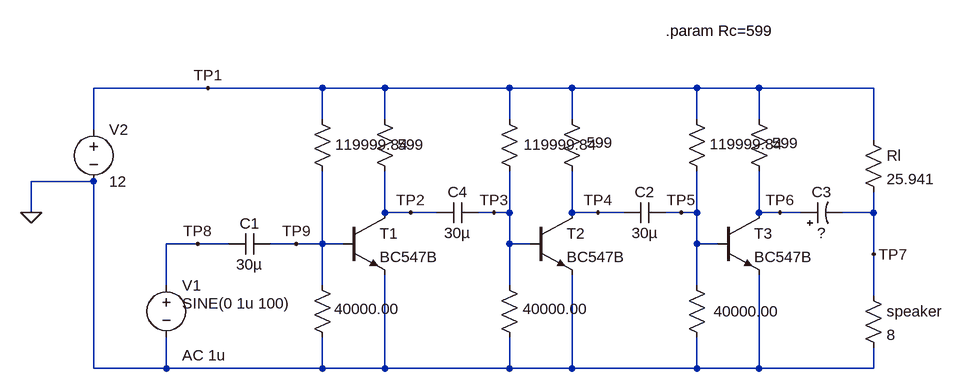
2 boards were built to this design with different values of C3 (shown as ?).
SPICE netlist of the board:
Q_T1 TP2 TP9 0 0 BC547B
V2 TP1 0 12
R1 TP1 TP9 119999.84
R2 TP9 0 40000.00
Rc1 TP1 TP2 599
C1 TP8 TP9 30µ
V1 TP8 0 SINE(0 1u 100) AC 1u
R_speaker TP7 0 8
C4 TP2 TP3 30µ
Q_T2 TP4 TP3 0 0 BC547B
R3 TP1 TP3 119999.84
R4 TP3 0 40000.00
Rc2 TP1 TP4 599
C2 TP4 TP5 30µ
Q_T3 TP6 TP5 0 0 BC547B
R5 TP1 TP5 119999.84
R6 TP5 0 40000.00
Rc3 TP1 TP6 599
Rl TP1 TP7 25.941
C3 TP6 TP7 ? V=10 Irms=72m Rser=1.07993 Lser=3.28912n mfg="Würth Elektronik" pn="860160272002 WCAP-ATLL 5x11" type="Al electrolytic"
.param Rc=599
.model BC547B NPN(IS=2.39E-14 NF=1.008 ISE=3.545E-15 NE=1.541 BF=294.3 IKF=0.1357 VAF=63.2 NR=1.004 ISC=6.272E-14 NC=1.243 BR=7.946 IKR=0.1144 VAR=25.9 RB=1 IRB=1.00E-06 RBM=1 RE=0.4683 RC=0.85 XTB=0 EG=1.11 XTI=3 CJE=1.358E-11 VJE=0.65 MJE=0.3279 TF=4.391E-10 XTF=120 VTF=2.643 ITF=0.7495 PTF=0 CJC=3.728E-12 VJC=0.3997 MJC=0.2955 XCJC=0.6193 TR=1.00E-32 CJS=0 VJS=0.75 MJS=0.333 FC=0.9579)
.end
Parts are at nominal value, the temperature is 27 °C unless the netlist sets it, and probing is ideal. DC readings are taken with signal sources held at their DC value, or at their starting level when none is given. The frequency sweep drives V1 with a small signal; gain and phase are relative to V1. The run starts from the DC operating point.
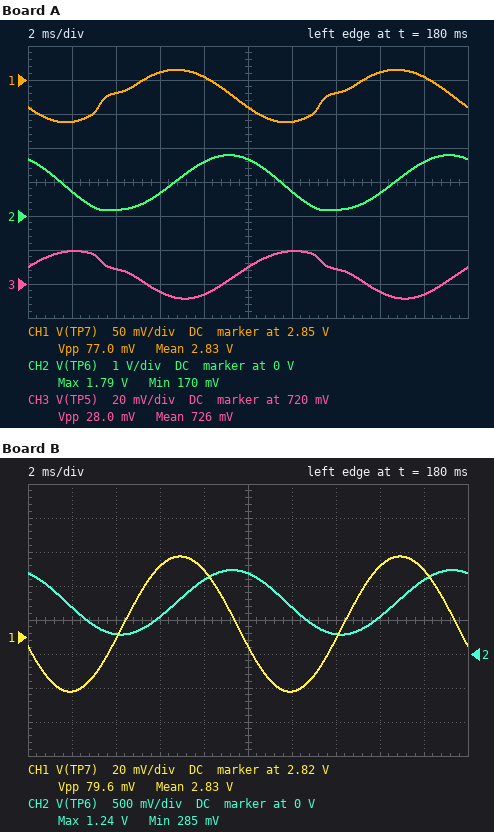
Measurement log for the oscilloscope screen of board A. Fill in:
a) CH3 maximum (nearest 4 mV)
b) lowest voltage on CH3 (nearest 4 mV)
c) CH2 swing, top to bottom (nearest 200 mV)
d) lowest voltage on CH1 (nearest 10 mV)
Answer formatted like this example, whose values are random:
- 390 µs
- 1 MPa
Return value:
- 740 mV
- 712 mV
- 1.6 V
- 2.79 V
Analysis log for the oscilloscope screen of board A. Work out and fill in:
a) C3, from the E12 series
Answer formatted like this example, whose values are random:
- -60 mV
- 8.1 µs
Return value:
- 12 µF
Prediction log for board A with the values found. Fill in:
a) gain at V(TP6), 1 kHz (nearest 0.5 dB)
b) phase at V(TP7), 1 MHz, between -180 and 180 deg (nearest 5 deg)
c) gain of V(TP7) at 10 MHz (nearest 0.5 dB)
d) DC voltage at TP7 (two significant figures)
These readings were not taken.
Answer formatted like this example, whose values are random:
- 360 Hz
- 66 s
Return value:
- 100.0 dB
- 110 deg
- 61.5 dB
- 2.8 V
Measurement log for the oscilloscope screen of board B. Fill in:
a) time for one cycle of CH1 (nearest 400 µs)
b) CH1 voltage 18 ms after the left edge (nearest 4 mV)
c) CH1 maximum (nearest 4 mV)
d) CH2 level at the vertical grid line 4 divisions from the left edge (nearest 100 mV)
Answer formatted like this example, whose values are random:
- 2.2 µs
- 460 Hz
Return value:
- 10.0 ms
- 2.860 V
- 2.868 V
- 1.1 V
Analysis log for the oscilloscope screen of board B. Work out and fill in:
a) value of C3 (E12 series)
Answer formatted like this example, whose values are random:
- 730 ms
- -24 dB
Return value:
- 22 µF
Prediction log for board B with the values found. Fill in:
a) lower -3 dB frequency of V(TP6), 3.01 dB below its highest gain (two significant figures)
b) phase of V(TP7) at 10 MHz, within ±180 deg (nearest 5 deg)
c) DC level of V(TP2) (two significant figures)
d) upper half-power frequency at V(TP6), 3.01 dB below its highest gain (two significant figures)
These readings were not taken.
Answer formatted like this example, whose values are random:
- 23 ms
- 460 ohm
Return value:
- 8.2 Hz
- 30 deg
- 690 mV
- 36 Hz
